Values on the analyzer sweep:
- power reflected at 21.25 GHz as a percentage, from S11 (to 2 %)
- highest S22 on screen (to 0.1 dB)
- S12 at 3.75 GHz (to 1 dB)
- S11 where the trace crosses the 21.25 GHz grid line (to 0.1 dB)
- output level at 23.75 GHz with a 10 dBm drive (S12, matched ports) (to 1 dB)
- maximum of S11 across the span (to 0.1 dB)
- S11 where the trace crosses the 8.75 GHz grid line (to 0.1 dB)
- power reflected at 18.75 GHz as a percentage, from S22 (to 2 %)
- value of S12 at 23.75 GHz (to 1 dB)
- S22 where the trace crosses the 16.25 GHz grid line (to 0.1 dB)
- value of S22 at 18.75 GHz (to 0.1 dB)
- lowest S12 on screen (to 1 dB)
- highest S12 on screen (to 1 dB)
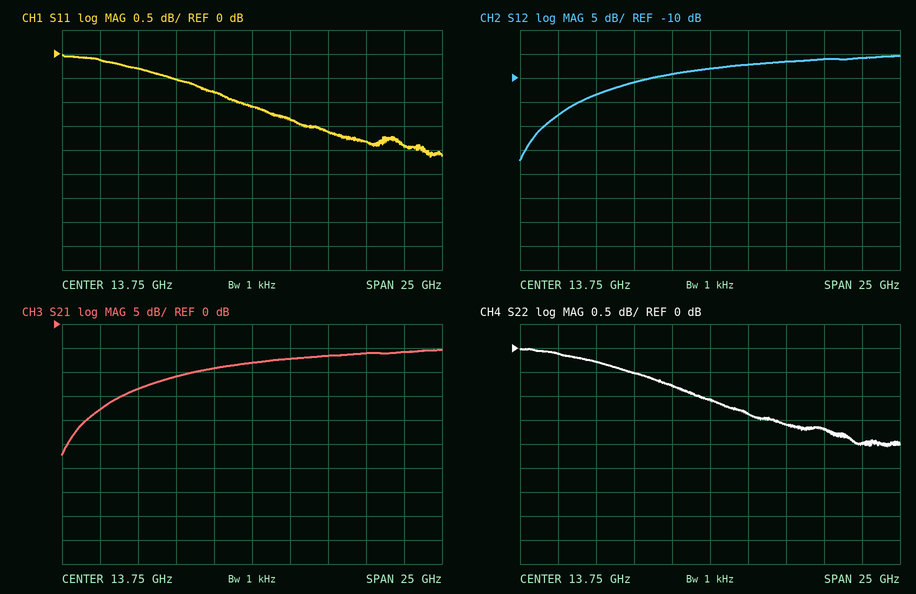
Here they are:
66 %
0.0 dB
-18 dB
-1.8 dB
4 dBm
0.0 dB
-0.5 dB
70 %
-6 dB
-1.4 dB
-1.6 dB
-27 dB
-5 dB
